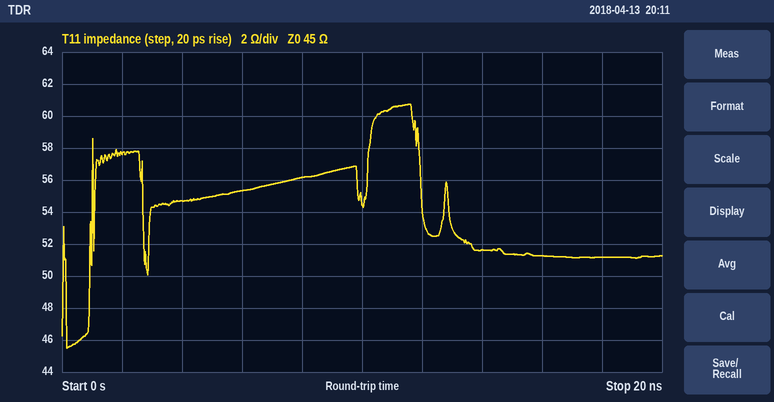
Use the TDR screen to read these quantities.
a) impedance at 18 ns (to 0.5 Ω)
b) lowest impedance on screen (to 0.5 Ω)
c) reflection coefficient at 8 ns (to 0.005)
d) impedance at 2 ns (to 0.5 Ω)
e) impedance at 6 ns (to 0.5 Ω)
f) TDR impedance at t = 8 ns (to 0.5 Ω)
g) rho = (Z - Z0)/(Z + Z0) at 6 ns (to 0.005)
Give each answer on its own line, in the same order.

51.0 Ω
45.5 Ω
+0.110
57.5 Ω
55.5 Ω
56.0 Ω
+0.105
